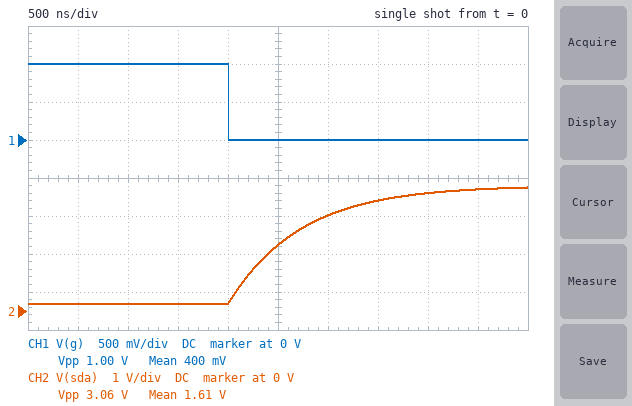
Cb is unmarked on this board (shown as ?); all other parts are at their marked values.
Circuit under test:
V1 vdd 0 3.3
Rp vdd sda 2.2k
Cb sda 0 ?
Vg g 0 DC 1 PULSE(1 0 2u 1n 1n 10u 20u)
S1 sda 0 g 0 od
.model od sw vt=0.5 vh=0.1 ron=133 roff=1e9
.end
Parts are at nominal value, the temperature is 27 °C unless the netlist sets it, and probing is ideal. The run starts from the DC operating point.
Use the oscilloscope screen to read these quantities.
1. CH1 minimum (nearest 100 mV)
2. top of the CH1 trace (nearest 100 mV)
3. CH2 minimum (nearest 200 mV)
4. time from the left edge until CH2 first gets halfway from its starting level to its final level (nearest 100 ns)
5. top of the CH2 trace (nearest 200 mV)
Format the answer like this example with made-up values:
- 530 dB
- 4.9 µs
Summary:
- 0 V
- 1.0 V
- 200 mV
- 2.5 µs
- 3.2 V
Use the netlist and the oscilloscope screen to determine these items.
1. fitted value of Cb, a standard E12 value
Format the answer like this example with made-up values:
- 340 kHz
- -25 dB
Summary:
- 330 pF
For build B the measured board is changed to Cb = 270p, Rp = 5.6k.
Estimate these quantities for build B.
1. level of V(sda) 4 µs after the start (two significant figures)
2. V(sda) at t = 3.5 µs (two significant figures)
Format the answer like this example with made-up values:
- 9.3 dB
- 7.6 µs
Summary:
- 2.4 V
- 2.1 V
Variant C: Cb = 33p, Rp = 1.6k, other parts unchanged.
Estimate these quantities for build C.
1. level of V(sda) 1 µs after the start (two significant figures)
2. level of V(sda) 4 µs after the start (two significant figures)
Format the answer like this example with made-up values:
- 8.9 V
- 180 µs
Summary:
- 250 mV
- 3.3 V
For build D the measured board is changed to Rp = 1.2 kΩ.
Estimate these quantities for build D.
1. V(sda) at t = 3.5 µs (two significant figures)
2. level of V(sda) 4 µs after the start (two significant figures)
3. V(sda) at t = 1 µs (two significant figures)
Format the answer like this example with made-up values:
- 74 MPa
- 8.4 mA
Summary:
- 3.2 V
- 3.3 V
- 330 mV
